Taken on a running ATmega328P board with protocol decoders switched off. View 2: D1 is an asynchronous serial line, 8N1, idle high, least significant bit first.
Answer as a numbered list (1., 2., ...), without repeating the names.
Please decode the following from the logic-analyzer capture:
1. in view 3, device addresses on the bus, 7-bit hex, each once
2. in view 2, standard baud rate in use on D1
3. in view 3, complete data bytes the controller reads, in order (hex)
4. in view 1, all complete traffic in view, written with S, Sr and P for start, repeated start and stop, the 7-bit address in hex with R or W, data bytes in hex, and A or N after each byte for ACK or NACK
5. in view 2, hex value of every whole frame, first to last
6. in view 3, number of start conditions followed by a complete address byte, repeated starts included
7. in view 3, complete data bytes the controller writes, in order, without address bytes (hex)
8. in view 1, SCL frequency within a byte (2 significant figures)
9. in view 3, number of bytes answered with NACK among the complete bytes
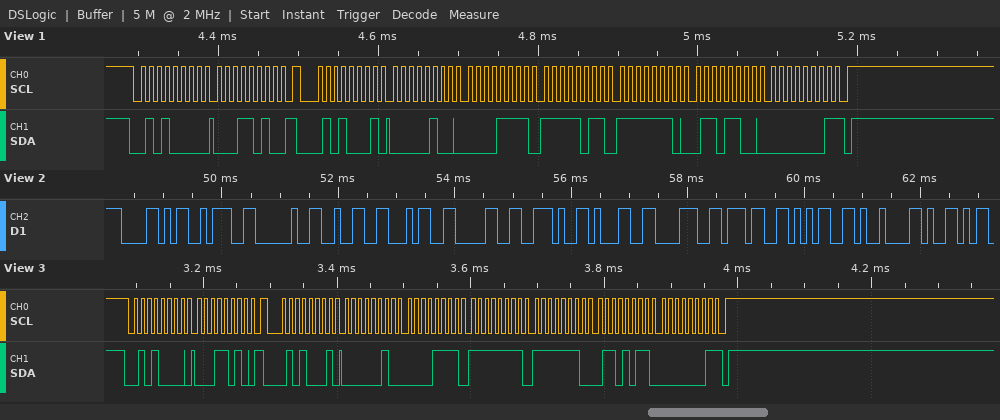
1. 0x28
2. 9600 baud
3. 02 0F FF FE 6B 01
4. S 28W A 1A A Sr 28R A 04 A 0F A FB A FE A 6C A 01 N P
5. 58 3A 20 32 34 30 2E 31 38 37 35 09 59
6. 2
7. 1A
8. 100 kHz
9. 1
